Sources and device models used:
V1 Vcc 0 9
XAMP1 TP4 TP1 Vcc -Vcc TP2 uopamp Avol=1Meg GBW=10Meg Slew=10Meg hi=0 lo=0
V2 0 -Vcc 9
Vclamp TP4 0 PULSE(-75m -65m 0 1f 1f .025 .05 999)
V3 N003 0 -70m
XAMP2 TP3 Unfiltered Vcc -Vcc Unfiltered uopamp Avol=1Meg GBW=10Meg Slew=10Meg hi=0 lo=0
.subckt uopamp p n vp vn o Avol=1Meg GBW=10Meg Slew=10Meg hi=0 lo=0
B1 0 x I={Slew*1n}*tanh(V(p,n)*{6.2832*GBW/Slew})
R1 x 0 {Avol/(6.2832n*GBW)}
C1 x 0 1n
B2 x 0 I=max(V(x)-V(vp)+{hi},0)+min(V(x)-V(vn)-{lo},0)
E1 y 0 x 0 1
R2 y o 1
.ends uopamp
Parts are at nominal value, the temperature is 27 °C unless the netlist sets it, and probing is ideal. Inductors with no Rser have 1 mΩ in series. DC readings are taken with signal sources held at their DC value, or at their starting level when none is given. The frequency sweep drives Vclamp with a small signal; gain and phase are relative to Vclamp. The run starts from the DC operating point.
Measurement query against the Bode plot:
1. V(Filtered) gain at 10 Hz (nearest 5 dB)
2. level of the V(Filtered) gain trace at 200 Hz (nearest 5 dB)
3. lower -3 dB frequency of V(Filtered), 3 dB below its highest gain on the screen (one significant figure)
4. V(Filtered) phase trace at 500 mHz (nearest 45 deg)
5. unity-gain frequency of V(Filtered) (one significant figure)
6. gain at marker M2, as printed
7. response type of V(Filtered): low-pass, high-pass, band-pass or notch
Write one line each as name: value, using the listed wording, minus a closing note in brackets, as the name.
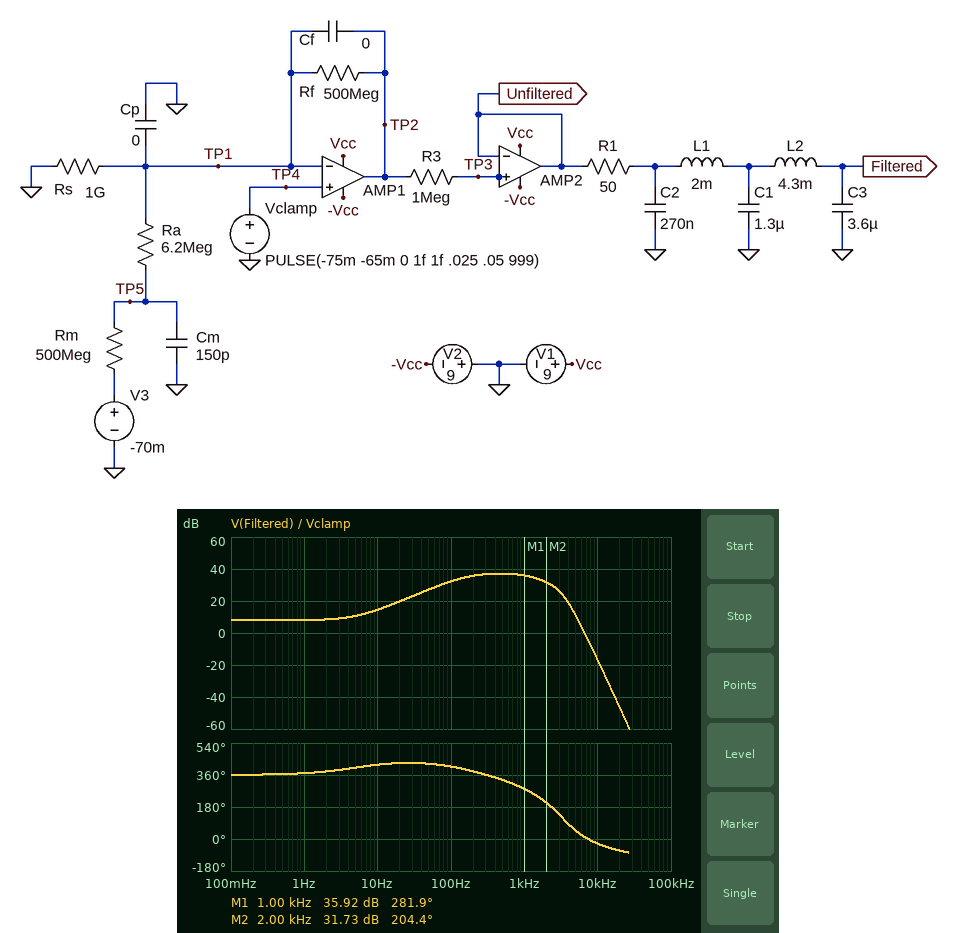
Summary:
V(Filtered) gain at 10 Hz: 15 dB
level of the V(Filtered) gain trace at 200 Hz: 35 dB
lower -3 dB frequency of V(Filtered), 3 dB below its highest gain on the screen: 100 Hz
V(Filtered) phase trace at 500 mHz: 360 deg
unity-gain frequency of V(Filtered): 7 kHz
gain at marker M2, as printed: 31.73 dB
response type of V(Filtered): low-pass, high-pass, band-pass or notch: band-pass
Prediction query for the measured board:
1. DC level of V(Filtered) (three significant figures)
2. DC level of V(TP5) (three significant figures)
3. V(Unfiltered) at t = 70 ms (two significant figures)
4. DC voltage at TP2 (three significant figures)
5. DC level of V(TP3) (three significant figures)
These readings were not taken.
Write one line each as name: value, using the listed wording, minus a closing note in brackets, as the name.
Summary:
DC level of V(Filtered): -117 mV
DC level of V(TP5): -74.9 mV
V(Unfiltered) at t = 70 ms: -93 mV
DC voltage at TP2: -117 mV
DC level of V(TP3): -117 mV
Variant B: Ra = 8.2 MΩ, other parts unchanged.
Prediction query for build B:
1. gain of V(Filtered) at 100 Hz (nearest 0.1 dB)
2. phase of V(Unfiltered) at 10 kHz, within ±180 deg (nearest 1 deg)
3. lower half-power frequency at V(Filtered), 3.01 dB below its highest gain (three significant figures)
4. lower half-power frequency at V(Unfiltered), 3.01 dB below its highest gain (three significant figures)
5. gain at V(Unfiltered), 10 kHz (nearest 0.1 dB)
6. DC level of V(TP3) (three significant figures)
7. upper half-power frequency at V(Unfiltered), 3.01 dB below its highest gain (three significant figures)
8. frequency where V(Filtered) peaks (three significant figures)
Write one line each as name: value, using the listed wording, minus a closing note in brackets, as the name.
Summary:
gain of V(Filtered) at 100 Hz: 31.5 dB
phase of V(Unfiltered) at 10 kHz, within ±180 deg: -3 deg
lower half-power frequency at V(Filtered), 3.01 dB below its highest gain: 110 Hz
lower half-power frequency at V(Unfiltered), 3.01 dB below its highest gain: 131 Hz
gain at V(Unfiltered), 10 kHz: 35.9 dB
DC level of V(TP3): -117 mV
upper half-power frequency at V(Unfiltered), 3.01 dB below its highest gain: 160 kHz
frequency where V(Filtered) peaks: 403 Hz
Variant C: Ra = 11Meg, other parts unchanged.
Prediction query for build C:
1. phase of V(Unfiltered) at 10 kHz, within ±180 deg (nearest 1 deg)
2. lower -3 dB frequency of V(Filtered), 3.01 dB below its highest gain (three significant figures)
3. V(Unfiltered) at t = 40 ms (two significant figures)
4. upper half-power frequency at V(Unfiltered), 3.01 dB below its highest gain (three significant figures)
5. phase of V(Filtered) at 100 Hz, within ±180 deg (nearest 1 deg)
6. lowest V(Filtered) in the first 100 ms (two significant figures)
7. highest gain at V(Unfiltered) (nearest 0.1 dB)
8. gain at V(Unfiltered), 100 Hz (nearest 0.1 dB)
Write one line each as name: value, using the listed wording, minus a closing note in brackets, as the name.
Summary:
phase of V(Unfiltered) at 10 kHz, within ±180 deg: -2 deg
lower -3 dB frequency of V(Filtered), 3.01 dB below its highest gain: 85.6 Hz
V(Unfiltered) at t = 40 ms: -120 mV
upper half-power frequency at V(Unfiltered), 3.01 dB below its highest gain: 213 kHz
phase of V(Filtered) at 100 Hz, within ±180 deg: 32 deg
lowest V(Filtered) in the first 100 ms: -480 mV
highest gain at V(Unfiltered): 33.4 dB
gain at V(Unfiltered), 100 Hz: 30.5 dB
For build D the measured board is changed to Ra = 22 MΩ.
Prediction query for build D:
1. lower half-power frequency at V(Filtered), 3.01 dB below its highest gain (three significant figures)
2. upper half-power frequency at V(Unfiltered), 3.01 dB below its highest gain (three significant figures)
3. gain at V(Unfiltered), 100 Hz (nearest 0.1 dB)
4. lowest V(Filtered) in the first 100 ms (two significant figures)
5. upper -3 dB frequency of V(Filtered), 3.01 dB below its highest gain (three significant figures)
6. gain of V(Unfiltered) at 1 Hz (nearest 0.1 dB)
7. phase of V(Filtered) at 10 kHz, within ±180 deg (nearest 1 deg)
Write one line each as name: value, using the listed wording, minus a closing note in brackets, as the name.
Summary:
lower half-power frequency at V(Filtered), 3.01 dB below its highest gain: 46.2 Hz
upper half-power frequency at V(Unfiltered), 3.01 dB below its highest gain: 412 kHz
gain at V(Unfiltered), 100 Hz: 26.7 dB
lowest V(Filtered) in the first 100 ms: -310 mV
upper -3 dB frequency of V(Filtered), 3.01 dB below its highest gain: 1.28 kHz
gain of V(Unfiltered) at 1 Hz: 8.0 dB
phase of V(Filtered) at 10 kHz, within ±180 deg: -23 deg
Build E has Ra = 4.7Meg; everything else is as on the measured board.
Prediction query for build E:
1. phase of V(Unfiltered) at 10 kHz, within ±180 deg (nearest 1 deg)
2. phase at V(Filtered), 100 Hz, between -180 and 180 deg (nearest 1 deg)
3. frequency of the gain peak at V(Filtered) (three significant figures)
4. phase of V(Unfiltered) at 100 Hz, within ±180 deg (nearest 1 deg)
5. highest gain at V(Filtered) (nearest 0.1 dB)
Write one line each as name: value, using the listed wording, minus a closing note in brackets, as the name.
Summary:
phase of V(Unfiltered) at 10 kHz, within ±180 deg: -5 deg
phase at V(Filtered), 100 Hz, between -180 and 180 deg: 54 deg
frequency of the gain peak at V(Filtered): 529 Hz
phase of V(Unfiltered) at 100 Hz, within ±180 deg: 63 deg
highest gain at V(Filtered): 39.2 dB
